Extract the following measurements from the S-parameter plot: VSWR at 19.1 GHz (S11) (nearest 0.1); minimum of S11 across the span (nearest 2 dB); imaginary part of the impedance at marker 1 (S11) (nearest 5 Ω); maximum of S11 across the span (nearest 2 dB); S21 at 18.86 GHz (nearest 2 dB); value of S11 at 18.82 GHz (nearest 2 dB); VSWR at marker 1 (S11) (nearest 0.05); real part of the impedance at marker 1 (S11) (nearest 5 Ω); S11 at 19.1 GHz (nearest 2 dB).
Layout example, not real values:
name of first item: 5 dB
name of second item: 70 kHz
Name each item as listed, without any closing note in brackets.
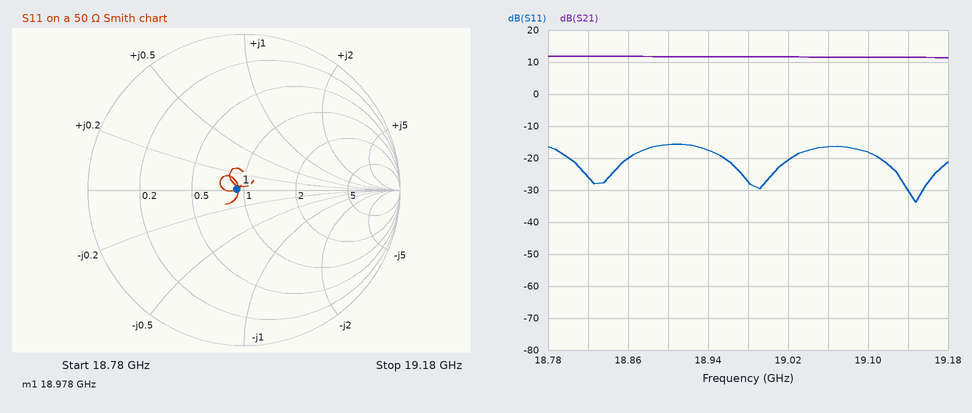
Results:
VSWR at 19.1 GHz (S11): 1.3
minimum of S11 across the span: -34 dB
imaginary part of the impedance at marker 1 (S11): 0 Ω
maximum of S11 across the span: -16 dB
S21 at 18.86 GHz: 12 dB
value of S11 at 18.82 GHz: -26 dB
VSWR at marker 1 (S11): 1.10
real part of the impedance at marker 1 (S11): 45 Ω
S11 at 19.1 GHz: -18 dB
